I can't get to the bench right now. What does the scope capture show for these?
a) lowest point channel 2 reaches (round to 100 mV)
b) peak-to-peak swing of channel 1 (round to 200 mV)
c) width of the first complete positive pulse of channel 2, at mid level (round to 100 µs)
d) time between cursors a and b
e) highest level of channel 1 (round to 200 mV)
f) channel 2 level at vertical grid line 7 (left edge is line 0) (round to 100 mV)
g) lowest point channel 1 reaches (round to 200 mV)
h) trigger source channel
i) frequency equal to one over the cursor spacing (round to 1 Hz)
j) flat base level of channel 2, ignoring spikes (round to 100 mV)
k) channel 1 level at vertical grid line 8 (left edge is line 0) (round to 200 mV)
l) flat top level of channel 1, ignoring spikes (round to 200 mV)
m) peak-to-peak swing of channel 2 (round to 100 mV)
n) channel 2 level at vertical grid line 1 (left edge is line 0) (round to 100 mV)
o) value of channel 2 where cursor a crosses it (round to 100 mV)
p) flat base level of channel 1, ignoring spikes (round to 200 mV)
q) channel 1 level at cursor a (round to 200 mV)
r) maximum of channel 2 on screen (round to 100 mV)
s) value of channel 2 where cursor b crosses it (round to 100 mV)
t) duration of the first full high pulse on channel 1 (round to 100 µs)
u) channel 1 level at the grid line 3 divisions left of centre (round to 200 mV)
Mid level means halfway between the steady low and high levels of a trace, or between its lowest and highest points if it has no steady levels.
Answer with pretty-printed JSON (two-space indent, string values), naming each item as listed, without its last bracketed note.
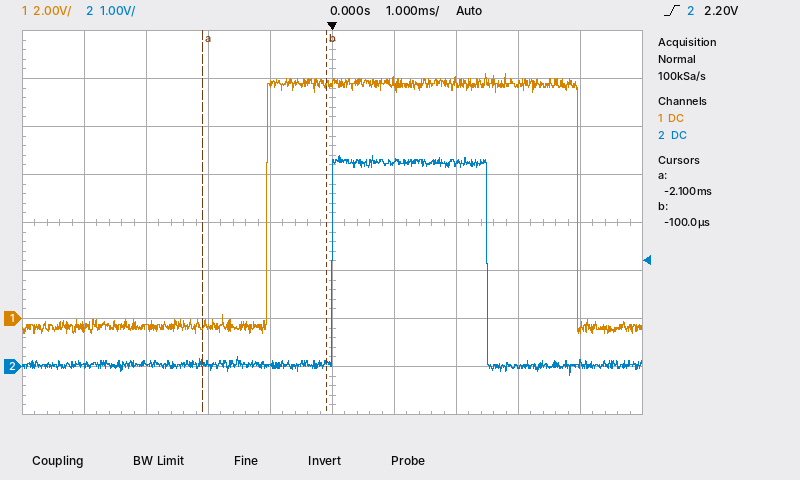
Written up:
{
  "lowest point channel 2 reaches": "-200 mV",
  "peak-to-peak swing of channel 1": "10.8 V",
  "width of the first complete positive pulse of channel 2, at mid level": "2.5 ms",
  "time between cursors a and b": "2.0 ms",
  "highest level of channel 1": "10.2 V",
  "channel 2 level at vertical grid line 7 (left edge is line 0)": "4.2 V",
  "lowest point channel 1 reaches": "-600 mV",
  "trigger source channel": "channel 2",
  "frequency equal to one over the cursor spacing": "500 Hz",
  "flat base level of channel 2, ignoring spikes": "0.0 V",
  "channel 1 level at vertical grid line 8 (left edge is line 0)": "9.8 V",
  "flat top level of channel 1, ignoring spikes": "9.8 V",
  "peak-to-peak swing of channel 2": "4.6 V",
  "channel 2 level at vertical grid line 1 (left edge is line 0)": "0.0 V",
  "value of channel 2 where cursor a crosses it": "100 mV",
  "flat base level of channel 1, ignoring spikes": "-400 mV",
  "channel 1 level at cursor a": "-200 mV",
  "maximum of channel 2 on screen": "4.4 V",
  "value of channel 2 where cursor b crosses it": "100 mV",
  "duration of the first full high pulse on channel 1": "5.0 ms",
  "channel 1 level at the grid line 3 divisions left of centre": "-400 mV"
}
